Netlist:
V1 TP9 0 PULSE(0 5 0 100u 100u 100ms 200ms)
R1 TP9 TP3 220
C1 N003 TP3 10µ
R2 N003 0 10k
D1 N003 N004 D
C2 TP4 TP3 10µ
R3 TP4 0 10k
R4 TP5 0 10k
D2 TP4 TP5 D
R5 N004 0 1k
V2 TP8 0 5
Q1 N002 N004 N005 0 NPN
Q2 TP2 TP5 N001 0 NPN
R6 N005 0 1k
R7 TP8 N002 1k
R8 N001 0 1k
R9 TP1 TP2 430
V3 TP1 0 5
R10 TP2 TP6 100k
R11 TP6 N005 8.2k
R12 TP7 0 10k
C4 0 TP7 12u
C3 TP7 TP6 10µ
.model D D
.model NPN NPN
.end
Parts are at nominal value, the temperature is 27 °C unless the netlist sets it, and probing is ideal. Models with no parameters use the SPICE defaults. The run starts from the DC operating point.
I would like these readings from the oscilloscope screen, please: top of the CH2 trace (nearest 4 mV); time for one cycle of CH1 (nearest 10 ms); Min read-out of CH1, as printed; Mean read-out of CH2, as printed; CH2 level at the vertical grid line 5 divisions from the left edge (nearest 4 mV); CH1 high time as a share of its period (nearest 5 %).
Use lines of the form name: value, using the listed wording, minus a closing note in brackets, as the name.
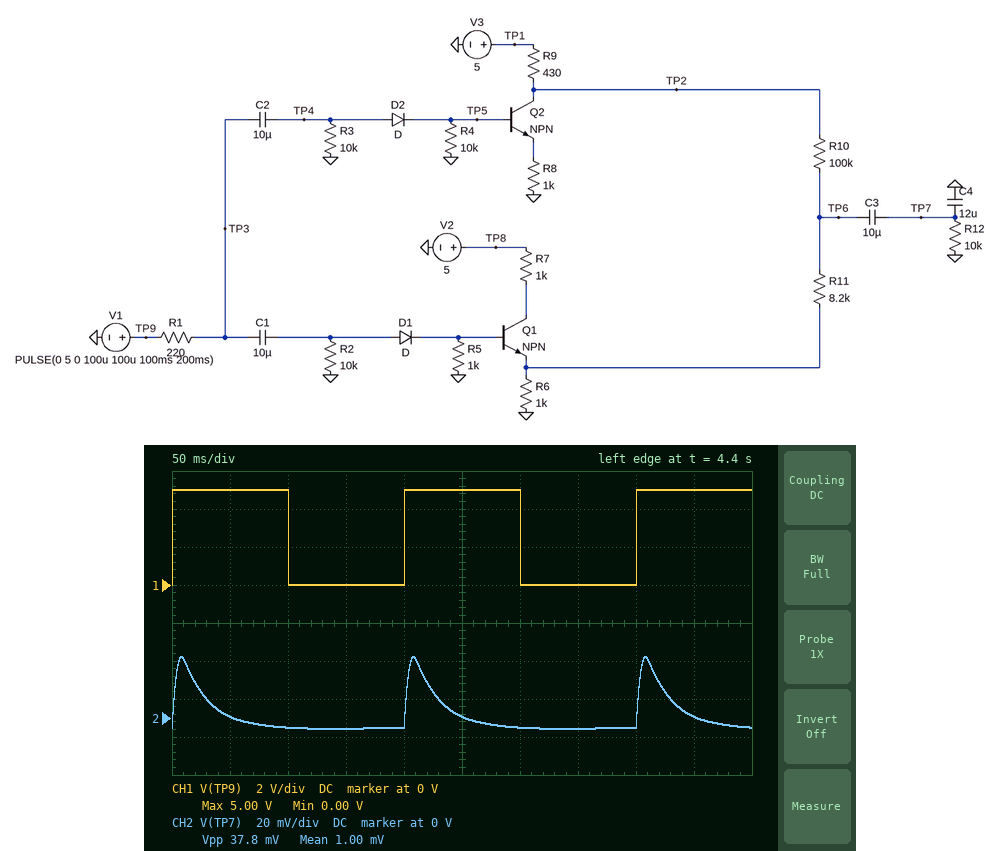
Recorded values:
top of the CH2 trace: 32 mV
time for one cycle of CH1: 200 ms
Min read-out of CH1, as printed: 0.00 V
Mean read-out of CH2, as printed: 1.00 mV
CH2 level at the vertical grid line 5 divisions from the left edge: 0 V
CH1 high time as a share of its period: 50 %
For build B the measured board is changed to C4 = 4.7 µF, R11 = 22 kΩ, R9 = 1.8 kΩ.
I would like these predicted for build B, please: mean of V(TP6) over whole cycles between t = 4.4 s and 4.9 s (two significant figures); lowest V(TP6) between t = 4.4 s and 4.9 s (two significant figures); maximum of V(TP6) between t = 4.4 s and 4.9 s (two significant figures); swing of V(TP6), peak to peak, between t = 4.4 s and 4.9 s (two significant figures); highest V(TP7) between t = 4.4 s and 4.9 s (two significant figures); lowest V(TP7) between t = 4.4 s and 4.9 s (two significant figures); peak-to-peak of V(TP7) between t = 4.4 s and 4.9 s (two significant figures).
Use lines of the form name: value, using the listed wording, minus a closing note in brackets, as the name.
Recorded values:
mean of V(TP6) over whole cycles between t = 4.4 s and 4.9 s: 880 mV
lowest V(TP6) between t = 4.4 s and 4.9 s: 830 mV
maximum of V(TP6) between t = 4.4 s and 4.9 s: 920 mV
swing of V(TP6), peak to peak, between t = 4.4 s and 4.9 s: 90 mV
highest V(TP7) between t = 4.4 s and 4.9 s: 22 mV
lowest V(TP7) between t = 4.4 s and 4.9 s: -36 mV
peak-to-peak of V(TP7) between t = 4.4 s and 4.9 s: 58 mV
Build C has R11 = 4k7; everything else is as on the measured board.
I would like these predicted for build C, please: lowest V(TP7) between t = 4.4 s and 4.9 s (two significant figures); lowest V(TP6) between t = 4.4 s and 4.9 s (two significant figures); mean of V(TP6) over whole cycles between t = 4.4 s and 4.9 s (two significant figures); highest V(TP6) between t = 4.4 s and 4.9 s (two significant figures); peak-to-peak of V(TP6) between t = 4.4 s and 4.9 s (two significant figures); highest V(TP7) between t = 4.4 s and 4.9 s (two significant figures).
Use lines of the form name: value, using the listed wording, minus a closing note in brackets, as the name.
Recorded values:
lowest V(TP7) between t = 4.4 s and 4.9 s: -8.5 mV
lowest V(TP6) between t = 4.4 s and 4.9 s: 270 mV
mean of V(TP6) over whole cycles between t = 4.4 s and 4.9 s: 290 mV
highest V(TP6) between t = 4.4 s and 4.9 s: 410 mV
peak-to-peak of V(TP6) between t = 4.4 s and 4.9 s: 140 mV
highest V(TP7) between t = 4.4 s and 4.9 s: 55 mV
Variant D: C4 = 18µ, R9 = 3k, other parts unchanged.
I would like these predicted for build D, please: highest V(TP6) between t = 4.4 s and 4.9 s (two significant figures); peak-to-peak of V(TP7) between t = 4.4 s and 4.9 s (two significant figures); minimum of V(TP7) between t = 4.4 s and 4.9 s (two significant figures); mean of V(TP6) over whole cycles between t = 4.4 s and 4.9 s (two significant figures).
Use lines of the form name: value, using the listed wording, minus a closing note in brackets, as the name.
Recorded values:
highest V(TP6) between t = 4.4 s and 4.9 s: 450 mV
peak-to-peak of V(TP7) between t = 4.4 s and 4.9 s: 33 mV
minimum of V(TP7) between t = 4.4 s and 4.9 s: -13 mV
mean of V(TP6) over whole cycles between t = 4.4 s and 4.9 s: 390 mV
